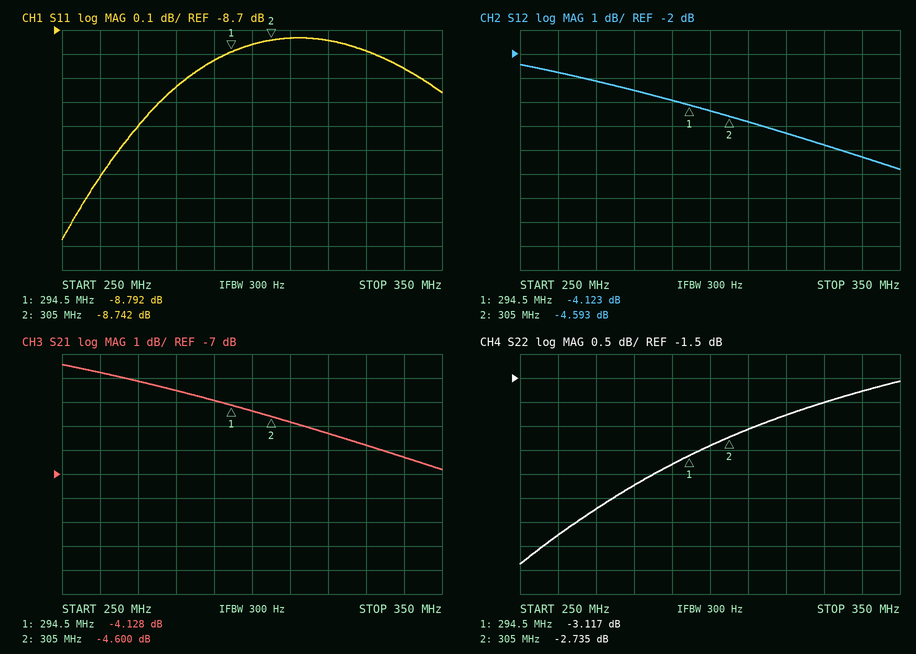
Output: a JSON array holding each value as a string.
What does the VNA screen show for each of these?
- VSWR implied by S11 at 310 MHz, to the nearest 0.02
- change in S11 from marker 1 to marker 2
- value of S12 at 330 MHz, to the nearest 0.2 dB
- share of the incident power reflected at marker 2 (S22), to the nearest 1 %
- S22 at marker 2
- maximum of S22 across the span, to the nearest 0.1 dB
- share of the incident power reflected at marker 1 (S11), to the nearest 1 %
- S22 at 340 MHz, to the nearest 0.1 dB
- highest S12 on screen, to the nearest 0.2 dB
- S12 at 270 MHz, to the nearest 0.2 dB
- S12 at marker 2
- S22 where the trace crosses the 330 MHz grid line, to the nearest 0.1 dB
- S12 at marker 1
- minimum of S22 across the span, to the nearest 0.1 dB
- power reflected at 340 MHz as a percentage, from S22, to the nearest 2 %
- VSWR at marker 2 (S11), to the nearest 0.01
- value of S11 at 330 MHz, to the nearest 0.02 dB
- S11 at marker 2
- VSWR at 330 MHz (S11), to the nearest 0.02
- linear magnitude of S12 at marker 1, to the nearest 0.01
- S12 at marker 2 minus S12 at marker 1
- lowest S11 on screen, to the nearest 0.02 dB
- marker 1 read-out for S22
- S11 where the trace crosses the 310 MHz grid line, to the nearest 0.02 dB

["2.16", "0.050 dB", "-5.8 dB", "53 %", "-2.735 dB", "-1.6 dB", "13 %", "-1.8 dB", "-2.4 dB", "-3.2 dB", "-4.593 dB", "-2.0 dB", "-4.123 dB", "-5.4 dB", "66 %", "2.15", "-8.78 dB", "-8.742 dB", "2.14", "0.62", "-0.470 dB", "-9.58 dB", "-3.117 dB", "-8.74 dB"]
